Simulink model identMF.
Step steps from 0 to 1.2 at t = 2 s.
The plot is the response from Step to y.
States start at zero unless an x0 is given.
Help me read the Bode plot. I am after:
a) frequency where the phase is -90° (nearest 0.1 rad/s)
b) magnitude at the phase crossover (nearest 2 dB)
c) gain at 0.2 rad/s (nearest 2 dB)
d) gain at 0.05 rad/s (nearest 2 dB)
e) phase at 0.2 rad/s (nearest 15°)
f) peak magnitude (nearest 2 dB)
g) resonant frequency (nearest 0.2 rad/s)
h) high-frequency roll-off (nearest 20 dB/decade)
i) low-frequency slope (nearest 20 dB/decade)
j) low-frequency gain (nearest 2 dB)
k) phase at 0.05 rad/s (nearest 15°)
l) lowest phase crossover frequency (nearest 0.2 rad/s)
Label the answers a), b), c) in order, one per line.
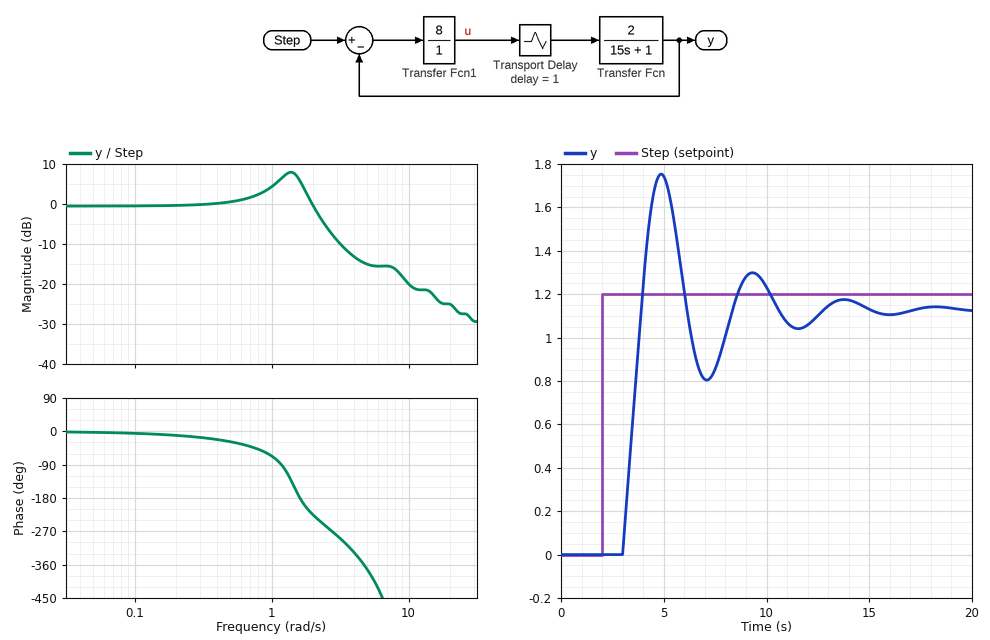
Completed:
a) 1.2 rad/s
b) 6 dB
c) 0 dB
d) 0 dB
e) -15°
f) 8 dB
g) 1.4 rad/s
h) -20 dB/decade
i) 0 dB/decade
j) 0 dB
k) 0°
l) 1.6 rad/s
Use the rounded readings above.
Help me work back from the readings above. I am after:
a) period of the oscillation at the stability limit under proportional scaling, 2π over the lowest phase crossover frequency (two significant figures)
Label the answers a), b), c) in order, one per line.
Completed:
a) 3.9 s
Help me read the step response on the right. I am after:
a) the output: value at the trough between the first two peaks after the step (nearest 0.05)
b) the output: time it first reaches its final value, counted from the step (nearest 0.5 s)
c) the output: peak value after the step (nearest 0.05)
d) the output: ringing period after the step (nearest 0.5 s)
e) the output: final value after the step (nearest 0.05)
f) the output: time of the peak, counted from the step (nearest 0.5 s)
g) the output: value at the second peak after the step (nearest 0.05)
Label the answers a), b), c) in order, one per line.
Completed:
a) 0.80
b) 2.0 s
c) 1.75
d) 4.5 s
e) 1.15
f) 3.0 s
g) 1.30
